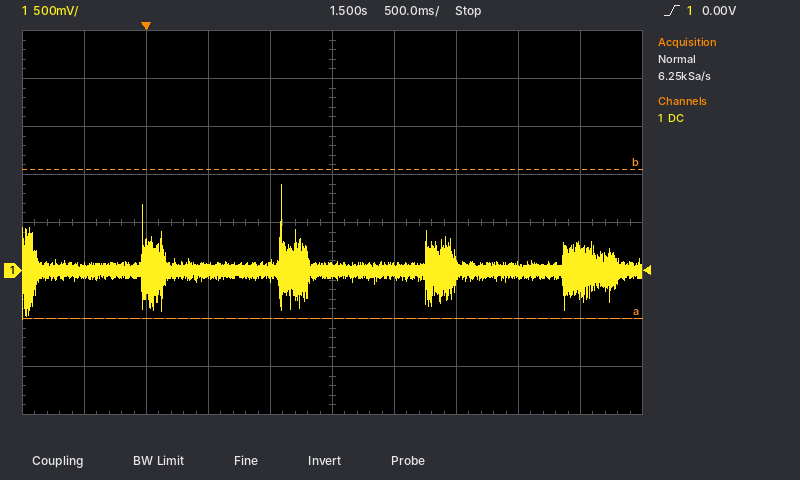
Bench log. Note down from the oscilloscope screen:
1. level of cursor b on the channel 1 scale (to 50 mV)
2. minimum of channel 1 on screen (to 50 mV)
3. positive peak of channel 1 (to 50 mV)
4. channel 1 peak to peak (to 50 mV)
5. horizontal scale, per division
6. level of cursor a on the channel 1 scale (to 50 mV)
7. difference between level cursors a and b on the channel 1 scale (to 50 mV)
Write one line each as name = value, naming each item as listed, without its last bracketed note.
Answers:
level of cursor b on the channel 1 scale = 1.05 V
minimum of channel 1 on screen = -500 mV
positive peak of channel 1 = 900 mV
channel 1 peak to peak = 1.40 V
horizontal scale, per division = 500 ms
level of cursor a on the channel 1 scale = -500 mV
difference between level cursors a and b on the channel 1 scale = 1.55 V
